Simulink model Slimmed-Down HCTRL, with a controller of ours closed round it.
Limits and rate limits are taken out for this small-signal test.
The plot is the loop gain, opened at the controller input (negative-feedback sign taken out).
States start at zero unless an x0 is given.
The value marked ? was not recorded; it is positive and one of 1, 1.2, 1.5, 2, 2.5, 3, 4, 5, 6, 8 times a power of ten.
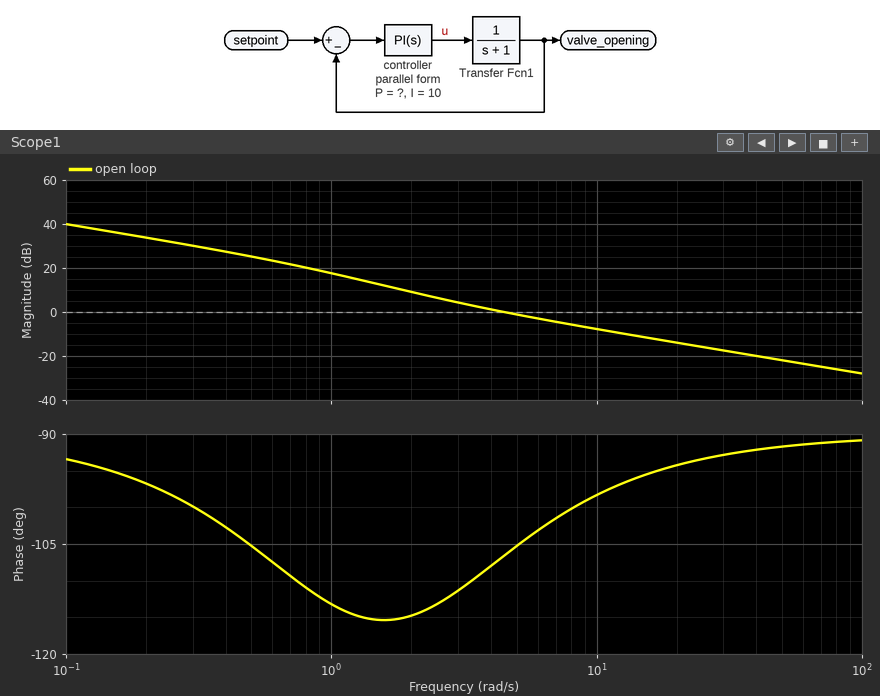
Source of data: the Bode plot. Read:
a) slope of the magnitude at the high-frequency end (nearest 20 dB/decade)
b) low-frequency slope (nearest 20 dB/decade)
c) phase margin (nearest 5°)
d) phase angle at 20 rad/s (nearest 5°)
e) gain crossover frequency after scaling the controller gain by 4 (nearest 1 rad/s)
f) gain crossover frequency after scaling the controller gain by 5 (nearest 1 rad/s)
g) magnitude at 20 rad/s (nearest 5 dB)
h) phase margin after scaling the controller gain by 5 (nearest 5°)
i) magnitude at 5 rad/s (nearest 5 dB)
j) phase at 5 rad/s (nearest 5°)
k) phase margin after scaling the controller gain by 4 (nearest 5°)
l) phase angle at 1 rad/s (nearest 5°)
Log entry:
-20 dB/decade
-20 dB/decade
75°
-95°
16 rad/s
20 rad/s
-15 dB
85°
0 dB
-105°
85°
-115°
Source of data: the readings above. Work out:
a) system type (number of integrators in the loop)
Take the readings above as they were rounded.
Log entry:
1
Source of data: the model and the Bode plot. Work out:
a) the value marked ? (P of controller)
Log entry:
4
